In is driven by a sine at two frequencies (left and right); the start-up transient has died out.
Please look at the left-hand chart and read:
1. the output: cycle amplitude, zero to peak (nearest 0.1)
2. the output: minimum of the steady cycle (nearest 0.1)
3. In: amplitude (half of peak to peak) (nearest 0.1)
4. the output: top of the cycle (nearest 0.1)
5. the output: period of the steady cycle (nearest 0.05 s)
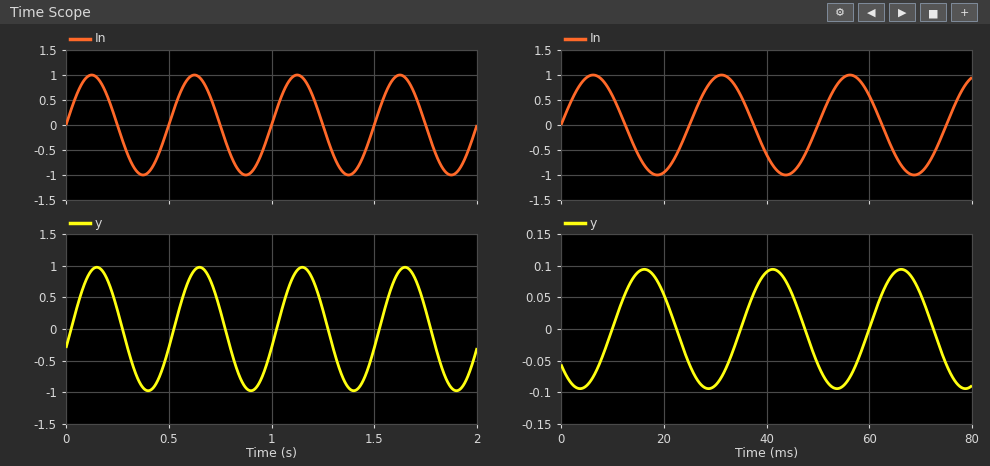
1.0
-1.0
1.0
1.0
0.50 s
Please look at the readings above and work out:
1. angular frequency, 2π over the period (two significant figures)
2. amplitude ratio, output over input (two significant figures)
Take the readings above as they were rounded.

13 rad/s
1.0
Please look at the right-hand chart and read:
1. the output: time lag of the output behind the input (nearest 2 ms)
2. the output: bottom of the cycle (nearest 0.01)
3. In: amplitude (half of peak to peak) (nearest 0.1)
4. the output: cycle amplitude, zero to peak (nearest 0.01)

10 ms
-0.09
1.0
0.09
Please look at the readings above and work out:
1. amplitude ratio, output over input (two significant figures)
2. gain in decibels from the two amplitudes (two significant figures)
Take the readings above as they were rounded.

0.090
-21 dB
